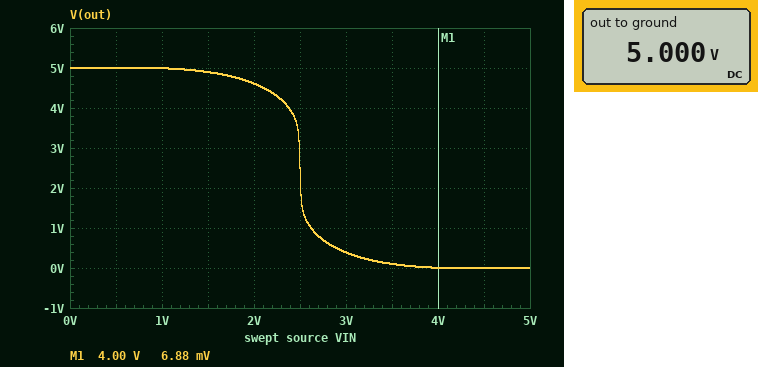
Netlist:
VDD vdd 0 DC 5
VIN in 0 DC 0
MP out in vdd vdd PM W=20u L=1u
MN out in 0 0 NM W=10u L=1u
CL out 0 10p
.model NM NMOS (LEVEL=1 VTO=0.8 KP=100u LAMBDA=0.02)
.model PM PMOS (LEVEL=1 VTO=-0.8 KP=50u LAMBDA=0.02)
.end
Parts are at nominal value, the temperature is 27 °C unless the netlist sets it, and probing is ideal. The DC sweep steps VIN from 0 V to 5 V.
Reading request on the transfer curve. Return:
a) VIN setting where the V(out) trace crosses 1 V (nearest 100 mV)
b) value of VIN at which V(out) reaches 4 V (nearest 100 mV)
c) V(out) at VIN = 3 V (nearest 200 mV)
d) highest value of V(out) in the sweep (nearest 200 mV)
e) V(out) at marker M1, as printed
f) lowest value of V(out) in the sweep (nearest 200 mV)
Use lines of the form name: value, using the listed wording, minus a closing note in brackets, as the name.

VIN setting where the V(out) trace crosses 1 V: 2.6 V
value of VIN at which V(out) reaches 4 V: 2.4 V
V(out) at VIN = 3 V: 400 mV
highest value of V(out) in the sweep: 5.0 V
V(out) at marker M1, as printed: 6.88 mV
lowest value of V(out) in the sweep: 0 V
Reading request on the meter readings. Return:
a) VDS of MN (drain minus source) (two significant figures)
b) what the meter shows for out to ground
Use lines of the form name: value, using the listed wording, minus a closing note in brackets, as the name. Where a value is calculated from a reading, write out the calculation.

VDS of MN (drain minus source): 5 V = 5.0 V
what the meter shows for out to ground: 5.000 V
